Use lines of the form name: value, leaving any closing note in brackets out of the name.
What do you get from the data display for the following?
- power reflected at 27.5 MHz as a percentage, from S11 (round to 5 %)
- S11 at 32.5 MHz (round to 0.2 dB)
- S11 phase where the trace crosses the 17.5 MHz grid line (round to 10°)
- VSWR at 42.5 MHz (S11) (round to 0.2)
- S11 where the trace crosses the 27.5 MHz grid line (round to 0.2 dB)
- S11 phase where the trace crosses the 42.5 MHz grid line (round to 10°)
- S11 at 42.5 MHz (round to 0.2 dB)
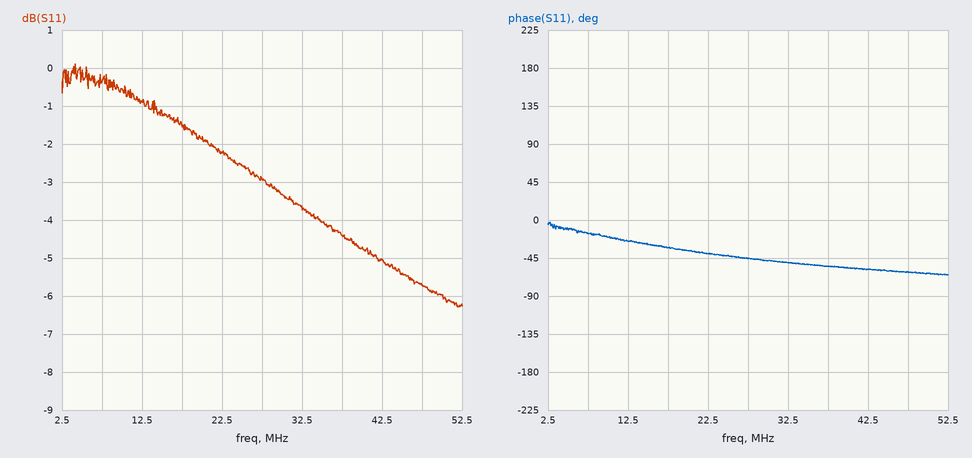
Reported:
power reflected at 27.5 MHz as a percentage, from S11: 50 %
S11 at 32.5 MHz: -3.6 dB
S11 phase where the trace crosses the 17.5 MHz grid line: -30°
VSWR at 42.5 MHz (S11): 3.6
S11 where the trace crosses the 27.5 MHz grid line: -3.0 dB
S11 phase where the trace crosses the 42.5 MHz grid line: -60°
S11 at 42.5 MHz: -5.0 dB
